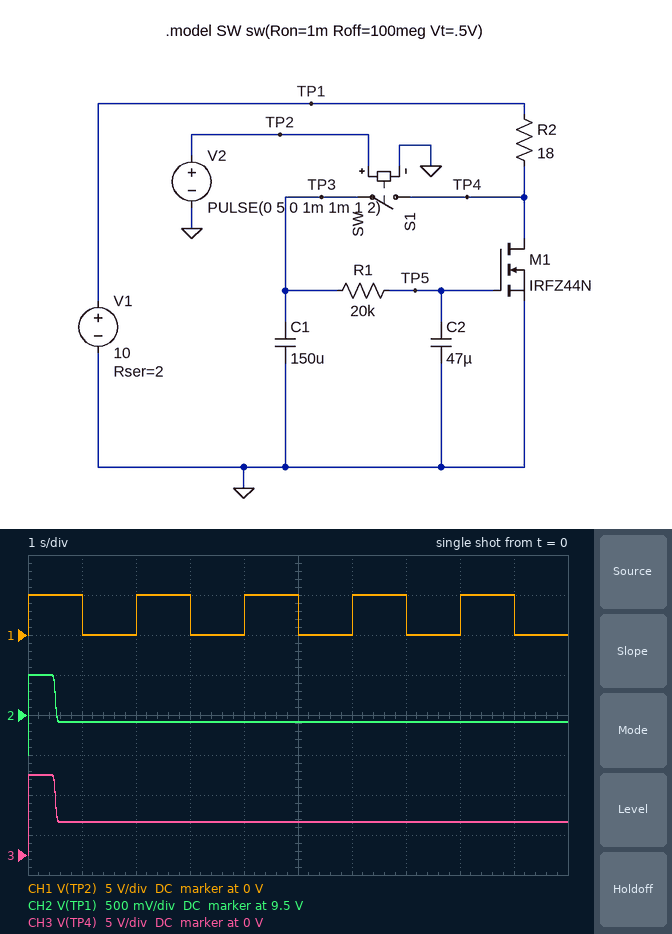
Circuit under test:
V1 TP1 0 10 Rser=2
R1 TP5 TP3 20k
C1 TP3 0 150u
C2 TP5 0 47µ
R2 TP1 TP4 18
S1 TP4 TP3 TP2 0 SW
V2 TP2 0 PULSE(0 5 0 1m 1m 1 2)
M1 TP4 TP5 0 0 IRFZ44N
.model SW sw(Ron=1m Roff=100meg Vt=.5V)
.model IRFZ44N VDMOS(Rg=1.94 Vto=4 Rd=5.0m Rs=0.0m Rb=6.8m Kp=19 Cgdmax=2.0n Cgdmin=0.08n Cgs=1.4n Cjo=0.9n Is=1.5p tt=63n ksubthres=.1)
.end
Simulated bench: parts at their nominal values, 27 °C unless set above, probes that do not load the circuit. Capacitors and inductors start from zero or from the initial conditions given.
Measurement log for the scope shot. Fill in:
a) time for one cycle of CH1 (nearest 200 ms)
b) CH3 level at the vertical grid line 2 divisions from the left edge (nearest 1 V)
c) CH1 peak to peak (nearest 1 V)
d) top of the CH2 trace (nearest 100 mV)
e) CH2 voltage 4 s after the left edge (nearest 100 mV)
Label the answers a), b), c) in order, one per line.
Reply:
a) 2.0 s
b) 4 V
c) 5 V
d) 10.0 V
e) 9.4 V
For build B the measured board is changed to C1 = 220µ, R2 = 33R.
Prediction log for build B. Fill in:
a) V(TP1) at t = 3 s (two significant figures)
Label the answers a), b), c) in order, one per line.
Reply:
a) 9.7 V
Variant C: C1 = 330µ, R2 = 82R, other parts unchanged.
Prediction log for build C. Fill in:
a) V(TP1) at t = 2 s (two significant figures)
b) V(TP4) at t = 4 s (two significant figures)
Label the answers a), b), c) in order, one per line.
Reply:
a) 9.9 V
b) 4.0 V
